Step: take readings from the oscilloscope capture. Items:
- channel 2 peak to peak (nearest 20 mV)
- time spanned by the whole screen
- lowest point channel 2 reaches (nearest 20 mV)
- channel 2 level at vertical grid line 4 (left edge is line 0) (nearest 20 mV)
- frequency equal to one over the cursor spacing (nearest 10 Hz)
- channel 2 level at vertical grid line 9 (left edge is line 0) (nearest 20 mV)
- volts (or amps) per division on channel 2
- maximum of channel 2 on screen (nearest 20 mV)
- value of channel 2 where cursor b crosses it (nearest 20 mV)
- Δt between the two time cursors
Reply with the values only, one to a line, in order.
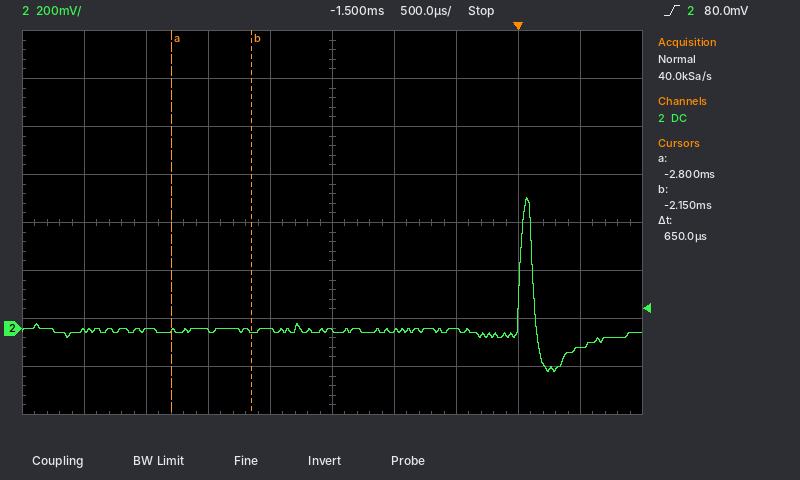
720 mV
5 ms
-180 mV
0 mV
1.54 kHz
-80 mV
200 mV
540 mV
-20 mV
650 µs
